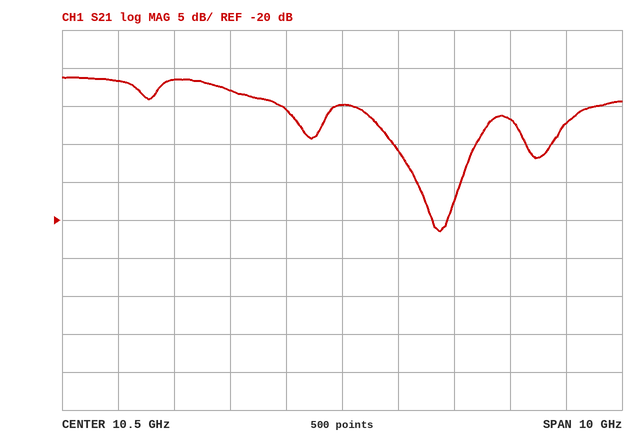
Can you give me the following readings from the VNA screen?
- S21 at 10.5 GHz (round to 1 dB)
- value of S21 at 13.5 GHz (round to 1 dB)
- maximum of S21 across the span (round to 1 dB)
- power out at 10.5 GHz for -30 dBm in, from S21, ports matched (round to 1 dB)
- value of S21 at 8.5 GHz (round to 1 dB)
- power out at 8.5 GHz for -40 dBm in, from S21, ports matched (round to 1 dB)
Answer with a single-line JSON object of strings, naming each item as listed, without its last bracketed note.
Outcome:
{"S21 at 10.5 GHz": "-5 dB", "value of S21 at 13.5 GHz": "-7 dB", "maximum of S21 across the span": "-1 dB", "power out at 10.5 GHz for -30 dBm in, from S21, ports matched": "-35 dBm", "value of S21 at 8.5 GHz": "-3 dB", "power out at 8.5 GHz for -40 dBm in, from S21, ports matched": "-43 dBm"}
